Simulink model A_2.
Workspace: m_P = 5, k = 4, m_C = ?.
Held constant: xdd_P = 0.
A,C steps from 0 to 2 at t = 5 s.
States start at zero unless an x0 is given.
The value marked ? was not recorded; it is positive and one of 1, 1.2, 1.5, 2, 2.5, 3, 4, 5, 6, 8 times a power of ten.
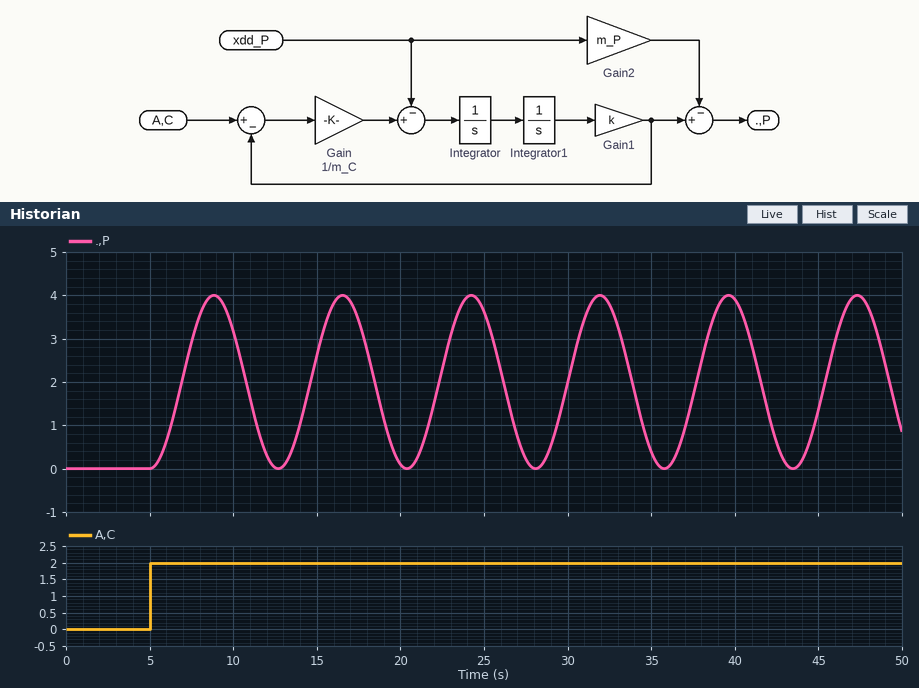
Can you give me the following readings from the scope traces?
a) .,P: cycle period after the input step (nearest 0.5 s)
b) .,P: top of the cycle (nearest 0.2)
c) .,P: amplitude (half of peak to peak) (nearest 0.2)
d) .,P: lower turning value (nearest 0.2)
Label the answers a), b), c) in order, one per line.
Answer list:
a) 7.5 s
b) 4.0
c) 2.0
d) 0.0
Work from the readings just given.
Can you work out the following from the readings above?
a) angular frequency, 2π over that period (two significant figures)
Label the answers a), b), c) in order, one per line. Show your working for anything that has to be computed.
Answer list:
a) 2π / 7.5 = 0.84 rad/s
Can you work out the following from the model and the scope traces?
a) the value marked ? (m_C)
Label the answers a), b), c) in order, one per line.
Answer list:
a) 6
